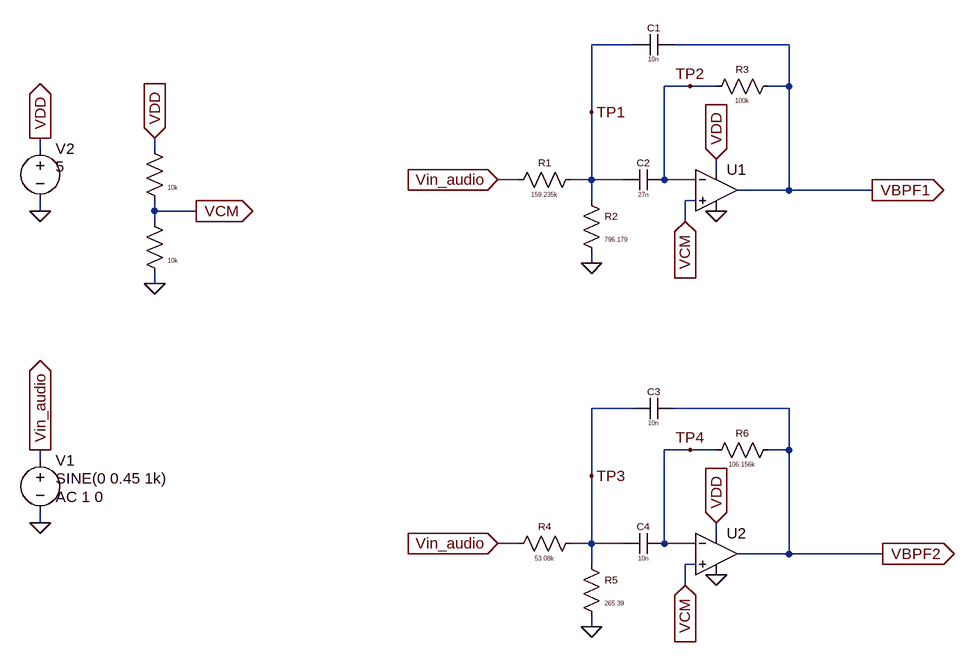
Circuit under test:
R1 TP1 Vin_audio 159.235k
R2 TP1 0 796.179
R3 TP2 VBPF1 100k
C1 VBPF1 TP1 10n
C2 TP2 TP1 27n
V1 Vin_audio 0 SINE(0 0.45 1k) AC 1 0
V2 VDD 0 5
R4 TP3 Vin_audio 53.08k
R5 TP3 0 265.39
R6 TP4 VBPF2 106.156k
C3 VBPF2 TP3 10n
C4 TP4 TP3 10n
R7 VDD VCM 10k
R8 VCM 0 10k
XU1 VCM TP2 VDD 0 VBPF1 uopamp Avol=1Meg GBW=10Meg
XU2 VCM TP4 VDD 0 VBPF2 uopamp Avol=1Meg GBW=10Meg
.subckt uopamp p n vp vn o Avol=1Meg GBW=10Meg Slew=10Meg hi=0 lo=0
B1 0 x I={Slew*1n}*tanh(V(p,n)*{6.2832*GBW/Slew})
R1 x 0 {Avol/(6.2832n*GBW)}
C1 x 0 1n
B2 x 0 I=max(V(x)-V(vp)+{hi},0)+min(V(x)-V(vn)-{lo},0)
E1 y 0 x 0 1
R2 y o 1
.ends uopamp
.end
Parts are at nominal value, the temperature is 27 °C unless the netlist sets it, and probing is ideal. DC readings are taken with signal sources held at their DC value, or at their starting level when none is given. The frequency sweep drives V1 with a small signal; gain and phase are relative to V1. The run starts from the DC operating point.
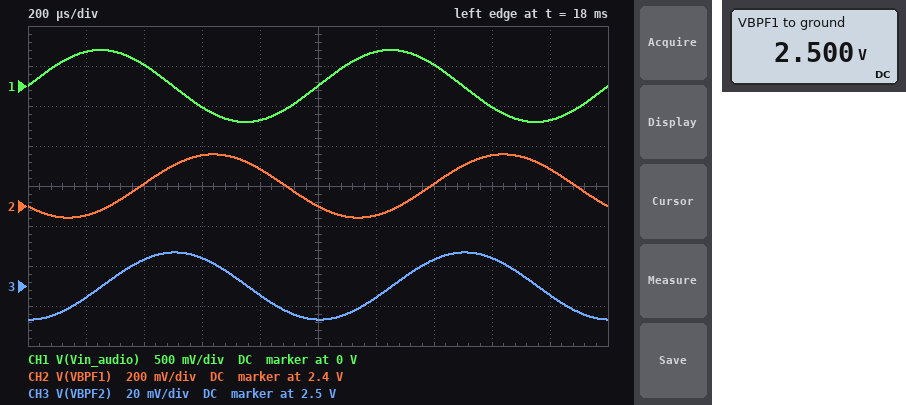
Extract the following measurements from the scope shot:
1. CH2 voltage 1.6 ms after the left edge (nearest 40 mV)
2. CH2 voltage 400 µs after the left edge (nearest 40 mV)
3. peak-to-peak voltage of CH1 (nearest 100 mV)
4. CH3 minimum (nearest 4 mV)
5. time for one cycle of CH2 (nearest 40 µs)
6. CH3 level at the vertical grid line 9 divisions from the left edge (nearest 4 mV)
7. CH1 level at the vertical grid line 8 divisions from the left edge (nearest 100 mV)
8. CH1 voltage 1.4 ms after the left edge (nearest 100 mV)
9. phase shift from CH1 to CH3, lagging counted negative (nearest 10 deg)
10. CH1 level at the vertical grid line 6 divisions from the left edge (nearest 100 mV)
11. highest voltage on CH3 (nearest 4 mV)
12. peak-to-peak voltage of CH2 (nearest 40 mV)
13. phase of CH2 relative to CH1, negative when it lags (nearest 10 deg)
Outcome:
2.64 V
2.52 V
900 mV
2.484 V
1.00 ms
2.496 V
-300 mV
300 mV
-90 deg
400 mV
2.516 V
320 mV
-140 deg
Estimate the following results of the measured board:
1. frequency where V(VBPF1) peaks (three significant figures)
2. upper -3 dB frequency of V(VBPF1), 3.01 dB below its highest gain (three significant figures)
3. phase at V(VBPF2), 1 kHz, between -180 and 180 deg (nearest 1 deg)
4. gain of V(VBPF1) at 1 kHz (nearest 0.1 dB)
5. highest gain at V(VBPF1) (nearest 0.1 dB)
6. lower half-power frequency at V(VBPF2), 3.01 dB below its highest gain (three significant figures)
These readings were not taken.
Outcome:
1.09 kHz
1.20 kHz
-92 deg
-9.1 dB
-6.8 dB
2.85 kHz
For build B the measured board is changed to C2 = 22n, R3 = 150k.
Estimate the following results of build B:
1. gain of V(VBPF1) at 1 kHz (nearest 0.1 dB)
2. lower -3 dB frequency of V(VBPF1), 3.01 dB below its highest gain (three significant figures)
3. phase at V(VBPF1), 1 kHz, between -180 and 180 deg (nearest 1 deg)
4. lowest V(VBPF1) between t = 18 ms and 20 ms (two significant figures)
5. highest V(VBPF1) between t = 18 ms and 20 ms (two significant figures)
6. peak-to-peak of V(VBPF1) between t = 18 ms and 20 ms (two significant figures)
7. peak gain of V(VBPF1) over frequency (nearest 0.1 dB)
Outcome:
-4.0 dB
909 Hz
168 deg
2.2 V
2.8 V
570 mV
-3.8 dB
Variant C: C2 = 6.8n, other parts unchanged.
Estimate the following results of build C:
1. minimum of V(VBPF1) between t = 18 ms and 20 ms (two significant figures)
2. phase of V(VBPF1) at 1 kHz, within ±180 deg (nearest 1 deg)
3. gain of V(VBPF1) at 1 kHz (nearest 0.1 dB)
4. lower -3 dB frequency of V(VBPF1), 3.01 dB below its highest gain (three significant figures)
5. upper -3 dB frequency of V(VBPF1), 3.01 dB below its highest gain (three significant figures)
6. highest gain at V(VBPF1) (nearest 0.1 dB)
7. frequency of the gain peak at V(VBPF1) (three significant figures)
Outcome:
2.5 V
-96 deg
-31.4 dB
1.98 kHz
2.37 kHz
-11.9 dB
2.17 kHz
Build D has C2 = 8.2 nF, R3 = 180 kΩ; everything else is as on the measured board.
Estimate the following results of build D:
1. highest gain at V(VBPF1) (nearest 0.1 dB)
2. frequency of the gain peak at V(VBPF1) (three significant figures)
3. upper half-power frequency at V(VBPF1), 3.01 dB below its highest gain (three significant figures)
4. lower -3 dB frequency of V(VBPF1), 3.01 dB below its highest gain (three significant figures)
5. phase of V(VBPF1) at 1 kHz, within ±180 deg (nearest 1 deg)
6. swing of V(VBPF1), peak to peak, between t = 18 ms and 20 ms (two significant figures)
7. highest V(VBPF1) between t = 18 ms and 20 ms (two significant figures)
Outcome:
-5.9 dB
1.47 kHz
1.57 kHz
1.38 kHz
-100 deg
76 mV
2.5 V
